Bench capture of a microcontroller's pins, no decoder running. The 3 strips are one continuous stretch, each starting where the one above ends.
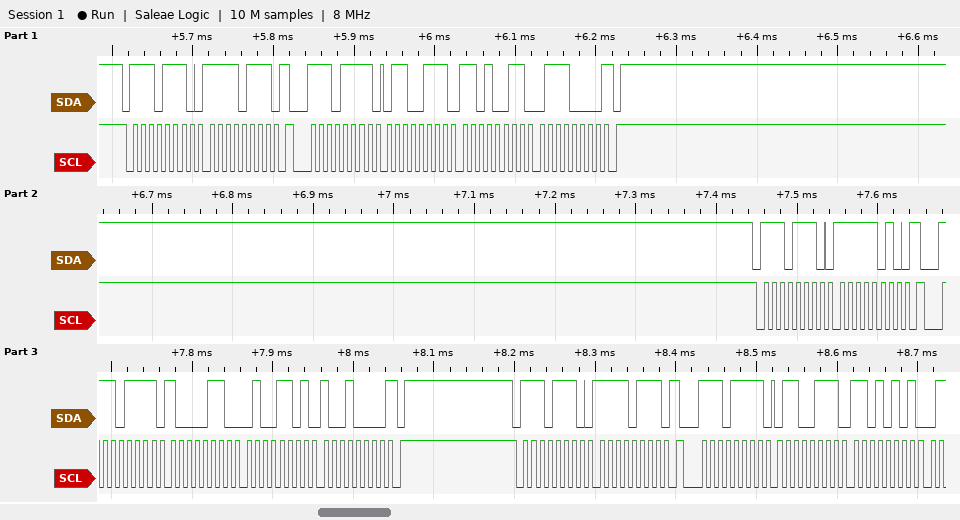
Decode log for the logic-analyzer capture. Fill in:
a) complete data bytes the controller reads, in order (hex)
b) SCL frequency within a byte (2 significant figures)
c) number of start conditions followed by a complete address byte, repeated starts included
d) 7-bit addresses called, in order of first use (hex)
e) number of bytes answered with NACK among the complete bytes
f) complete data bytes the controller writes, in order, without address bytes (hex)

67 D3 70 86 4D 90 67 D5
100 kHz
6
0x77
2
F7 FA F7
